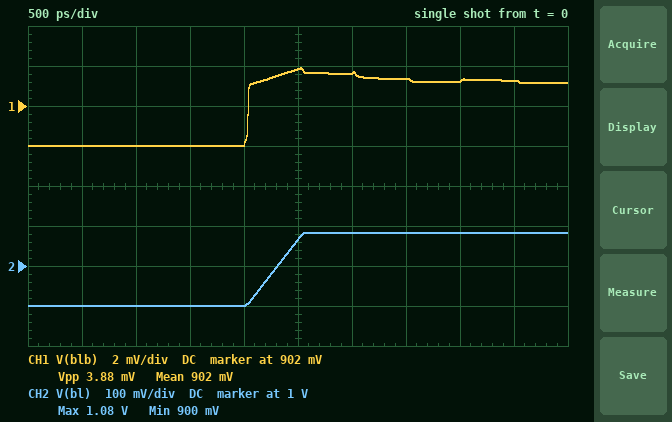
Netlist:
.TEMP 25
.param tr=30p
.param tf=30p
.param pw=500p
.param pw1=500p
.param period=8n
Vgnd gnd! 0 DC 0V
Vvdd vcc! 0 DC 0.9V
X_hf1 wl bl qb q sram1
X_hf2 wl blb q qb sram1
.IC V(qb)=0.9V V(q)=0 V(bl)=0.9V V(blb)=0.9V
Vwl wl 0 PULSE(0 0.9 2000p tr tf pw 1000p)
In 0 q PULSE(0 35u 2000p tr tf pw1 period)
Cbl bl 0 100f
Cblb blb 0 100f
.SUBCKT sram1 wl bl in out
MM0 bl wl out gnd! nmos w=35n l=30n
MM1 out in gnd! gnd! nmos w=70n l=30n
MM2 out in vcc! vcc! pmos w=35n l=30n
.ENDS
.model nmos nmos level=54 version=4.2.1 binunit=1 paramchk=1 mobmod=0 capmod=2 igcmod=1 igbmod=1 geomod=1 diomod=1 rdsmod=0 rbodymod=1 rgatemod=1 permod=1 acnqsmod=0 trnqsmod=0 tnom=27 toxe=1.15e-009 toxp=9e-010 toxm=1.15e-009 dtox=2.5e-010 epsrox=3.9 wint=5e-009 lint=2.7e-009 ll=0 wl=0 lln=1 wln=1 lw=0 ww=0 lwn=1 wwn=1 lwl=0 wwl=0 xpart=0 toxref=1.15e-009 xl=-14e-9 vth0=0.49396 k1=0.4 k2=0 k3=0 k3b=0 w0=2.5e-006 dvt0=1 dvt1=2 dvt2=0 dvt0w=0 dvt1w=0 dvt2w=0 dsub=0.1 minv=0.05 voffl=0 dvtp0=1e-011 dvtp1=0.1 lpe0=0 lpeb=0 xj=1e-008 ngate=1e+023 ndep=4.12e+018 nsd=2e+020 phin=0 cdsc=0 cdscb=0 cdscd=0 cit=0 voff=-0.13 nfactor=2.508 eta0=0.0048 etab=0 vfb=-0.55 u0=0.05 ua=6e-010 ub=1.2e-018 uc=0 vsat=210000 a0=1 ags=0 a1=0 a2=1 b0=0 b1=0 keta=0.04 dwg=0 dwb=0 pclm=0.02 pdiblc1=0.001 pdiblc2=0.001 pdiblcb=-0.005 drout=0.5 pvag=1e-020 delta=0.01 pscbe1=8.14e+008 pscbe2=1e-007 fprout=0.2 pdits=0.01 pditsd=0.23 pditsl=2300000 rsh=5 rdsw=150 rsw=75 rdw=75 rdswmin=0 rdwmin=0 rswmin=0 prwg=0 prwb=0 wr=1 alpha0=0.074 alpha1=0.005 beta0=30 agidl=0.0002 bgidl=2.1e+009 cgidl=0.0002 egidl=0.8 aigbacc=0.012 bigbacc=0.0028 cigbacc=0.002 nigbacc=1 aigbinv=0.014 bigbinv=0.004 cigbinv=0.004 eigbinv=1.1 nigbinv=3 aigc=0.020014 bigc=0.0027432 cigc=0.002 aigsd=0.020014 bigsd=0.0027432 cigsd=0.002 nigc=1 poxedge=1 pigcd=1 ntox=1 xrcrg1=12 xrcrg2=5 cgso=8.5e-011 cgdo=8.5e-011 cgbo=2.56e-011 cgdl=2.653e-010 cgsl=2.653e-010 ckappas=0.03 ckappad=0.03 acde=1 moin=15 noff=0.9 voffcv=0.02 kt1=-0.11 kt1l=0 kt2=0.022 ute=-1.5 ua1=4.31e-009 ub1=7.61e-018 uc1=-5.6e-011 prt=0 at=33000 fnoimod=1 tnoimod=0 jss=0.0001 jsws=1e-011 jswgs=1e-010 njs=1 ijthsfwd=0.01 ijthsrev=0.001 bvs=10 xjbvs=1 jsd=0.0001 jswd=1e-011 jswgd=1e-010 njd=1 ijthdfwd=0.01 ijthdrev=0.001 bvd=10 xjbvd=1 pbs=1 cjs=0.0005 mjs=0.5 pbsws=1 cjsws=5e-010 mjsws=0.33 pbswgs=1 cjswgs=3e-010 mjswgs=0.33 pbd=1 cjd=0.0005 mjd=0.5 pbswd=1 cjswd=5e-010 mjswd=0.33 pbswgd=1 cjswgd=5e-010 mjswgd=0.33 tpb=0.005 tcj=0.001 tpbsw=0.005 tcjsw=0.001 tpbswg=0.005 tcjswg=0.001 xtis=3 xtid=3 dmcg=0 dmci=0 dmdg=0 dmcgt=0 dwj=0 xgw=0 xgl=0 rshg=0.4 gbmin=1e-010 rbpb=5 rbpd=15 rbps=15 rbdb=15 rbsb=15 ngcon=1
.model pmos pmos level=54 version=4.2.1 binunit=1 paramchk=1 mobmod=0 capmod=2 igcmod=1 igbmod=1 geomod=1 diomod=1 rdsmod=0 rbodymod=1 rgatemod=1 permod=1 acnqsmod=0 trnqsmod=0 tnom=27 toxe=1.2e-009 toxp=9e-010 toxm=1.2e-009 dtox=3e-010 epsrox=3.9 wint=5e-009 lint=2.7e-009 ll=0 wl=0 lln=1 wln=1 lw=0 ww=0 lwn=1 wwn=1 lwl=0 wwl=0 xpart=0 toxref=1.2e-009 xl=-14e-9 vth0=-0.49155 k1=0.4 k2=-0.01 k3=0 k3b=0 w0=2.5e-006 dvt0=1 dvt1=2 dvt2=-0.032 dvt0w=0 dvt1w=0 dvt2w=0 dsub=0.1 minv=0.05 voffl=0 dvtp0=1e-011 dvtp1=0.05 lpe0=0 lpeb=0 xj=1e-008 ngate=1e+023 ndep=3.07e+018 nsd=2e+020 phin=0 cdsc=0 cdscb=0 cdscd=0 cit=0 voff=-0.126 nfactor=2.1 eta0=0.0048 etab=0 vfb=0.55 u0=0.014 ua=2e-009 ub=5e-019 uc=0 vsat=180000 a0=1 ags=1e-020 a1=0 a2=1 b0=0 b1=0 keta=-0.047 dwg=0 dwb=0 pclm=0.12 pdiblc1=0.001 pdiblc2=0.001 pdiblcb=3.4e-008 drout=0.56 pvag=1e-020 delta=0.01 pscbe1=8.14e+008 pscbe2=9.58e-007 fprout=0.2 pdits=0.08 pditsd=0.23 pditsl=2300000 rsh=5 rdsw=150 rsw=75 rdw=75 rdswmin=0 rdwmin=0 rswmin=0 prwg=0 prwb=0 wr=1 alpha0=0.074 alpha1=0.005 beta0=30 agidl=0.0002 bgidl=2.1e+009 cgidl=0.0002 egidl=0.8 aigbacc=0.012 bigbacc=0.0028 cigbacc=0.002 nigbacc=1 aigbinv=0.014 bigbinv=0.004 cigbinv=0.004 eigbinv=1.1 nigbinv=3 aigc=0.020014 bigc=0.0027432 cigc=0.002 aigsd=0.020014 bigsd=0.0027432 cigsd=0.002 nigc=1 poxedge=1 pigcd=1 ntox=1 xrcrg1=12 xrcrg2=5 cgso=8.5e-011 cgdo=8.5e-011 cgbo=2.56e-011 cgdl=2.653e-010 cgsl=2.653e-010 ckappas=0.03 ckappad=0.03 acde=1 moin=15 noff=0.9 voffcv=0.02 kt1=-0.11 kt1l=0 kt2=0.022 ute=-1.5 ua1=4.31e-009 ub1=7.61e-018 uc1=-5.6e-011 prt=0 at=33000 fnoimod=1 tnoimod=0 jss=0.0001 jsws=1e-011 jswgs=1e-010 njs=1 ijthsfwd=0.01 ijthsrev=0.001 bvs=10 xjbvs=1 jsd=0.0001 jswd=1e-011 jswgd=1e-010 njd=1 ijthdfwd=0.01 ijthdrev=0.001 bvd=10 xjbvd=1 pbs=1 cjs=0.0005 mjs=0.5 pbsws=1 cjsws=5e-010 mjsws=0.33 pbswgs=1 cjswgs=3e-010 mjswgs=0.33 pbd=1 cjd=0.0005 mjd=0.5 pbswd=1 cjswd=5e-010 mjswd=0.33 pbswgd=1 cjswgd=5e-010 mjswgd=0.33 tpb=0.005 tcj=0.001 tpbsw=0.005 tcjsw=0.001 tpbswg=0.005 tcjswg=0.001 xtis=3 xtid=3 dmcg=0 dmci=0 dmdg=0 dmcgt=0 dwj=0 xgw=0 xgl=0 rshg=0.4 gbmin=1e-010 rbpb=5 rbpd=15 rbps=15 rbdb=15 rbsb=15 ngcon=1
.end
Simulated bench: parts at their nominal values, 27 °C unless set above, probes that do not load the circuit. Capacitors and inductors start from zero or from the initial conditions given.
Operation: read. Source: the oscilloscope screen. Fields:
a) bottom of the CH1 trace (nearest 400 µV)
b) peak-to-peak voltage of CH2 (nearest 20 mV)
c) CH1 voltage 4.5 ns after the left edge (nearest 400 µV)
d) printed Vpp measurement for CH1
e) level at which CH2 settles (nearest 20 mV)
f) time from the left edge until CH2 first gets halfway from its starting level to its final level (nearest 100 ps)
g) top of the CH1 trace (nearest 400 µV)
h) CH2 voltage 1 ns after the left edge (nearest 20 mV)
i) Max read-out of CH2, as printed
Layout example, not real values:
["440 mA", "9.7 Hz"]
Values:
["900.0 mV", "180 mV", "903.2 mV", "3.88 mV", "1.08 V", "2.3 ns", "904.0 mV", "900 mV", "1.08 V"]
